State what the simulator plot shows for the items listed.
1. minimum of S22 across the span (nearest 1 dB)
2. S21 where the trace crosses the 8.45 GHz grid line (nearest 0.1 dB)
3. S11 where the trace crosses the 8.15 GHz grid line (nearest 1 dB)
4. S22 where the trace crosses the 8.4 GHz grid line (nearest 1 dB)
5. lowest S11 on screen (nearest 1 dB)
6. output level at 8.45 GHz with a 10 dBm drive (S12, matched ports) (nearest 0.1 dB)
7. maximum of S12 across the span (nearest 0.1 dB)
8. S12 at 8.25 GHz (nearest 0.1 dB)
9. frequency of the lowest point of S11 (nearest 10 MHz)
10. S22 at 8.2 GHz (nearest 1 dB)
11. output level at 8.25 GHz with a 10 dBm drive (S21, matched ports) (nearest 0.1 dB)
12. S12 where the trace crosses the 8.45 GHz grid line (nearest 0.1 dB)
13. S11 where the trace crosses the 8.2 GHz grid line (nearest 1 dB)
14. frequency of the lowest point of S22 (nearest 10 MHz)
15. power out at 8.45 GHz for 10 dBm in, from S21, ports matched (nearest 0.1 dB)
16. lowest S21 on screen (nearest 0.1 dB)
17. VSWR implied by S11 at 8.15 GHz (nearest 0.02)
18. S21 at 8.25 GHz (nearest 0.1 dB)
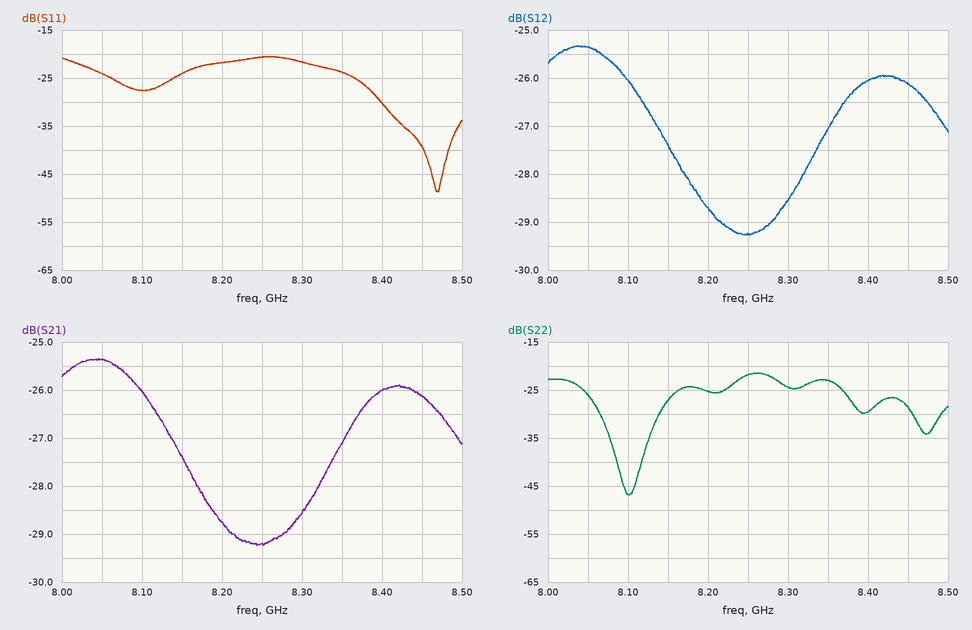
-47 dB
-26.1 dB
-24 dB
-30 dB
-49 dB
-16.1 dBm
-25.3 dB
-29.2 dB
8.47 GHz
-25 dB
-19.2 dBm
-26.1 dB
-22 dB
8.10 GHz
-16.1 dBm
-29.2 dB
1.14
-29.2 dB
